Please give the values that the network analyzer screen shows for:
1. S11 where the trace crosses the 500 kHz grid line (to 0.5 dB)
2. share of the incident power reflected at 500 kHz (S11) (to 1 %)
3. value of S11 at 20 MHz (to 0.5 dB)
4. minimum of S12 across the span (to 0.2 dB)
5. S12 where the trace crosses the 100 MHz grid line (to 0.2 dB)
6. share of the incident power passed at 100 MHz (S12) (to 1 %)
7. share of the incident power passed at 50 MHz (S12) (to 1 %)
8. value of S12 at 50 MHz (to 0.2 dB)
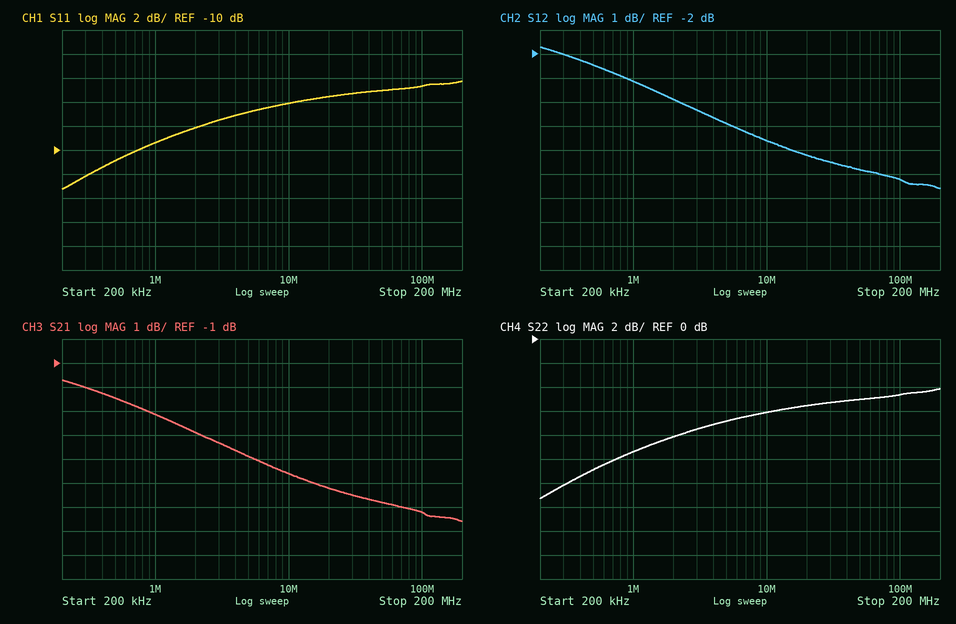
-11.0 dB
8 %
-5.5 dB
-7.6 dB
-7.2 dB
19 %
21 %
-6.8 dB
